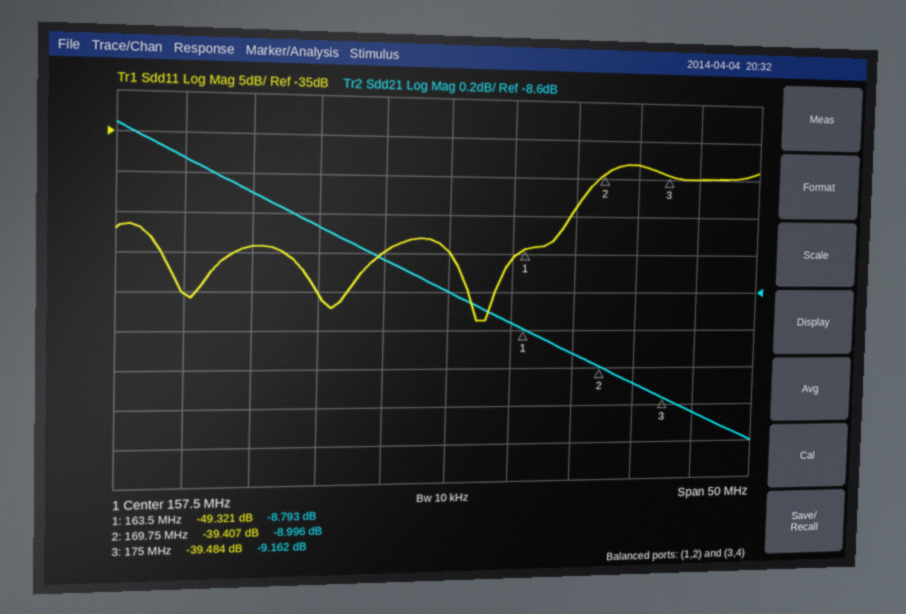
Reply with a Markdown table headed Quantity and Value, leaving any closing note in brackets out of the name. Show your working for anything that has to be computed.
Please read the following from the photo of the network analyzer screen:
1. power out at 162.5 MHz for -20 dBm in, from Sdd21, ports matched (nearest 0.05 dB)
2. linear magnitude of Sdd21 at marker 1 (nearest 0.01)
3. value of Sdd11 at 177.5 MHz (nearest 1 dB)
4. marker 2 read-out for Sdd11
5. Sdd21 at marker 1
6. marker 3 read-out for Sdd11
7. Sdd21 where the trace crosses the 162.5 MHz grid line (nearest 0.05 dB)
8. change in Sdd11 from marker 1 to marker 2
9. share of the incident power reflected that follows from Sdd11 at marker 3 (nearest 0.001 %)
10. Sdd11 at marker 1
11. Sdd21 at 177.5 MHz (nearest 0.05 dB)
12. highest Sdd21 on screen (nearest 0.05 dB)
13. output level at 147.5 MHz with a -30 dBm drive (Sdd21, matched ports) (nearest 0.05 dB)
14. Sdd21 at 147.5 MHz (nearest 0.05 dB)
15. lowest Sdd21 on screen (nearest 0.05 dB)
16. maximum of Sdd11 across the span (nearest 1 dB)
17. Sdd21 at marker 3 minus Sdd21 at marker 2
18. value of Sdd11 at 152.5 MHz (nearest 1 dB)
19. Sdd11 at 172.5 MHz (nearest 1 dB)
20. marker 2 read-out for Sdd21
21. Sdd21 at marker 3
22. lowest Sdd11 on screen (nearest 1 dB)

| Quantity | Value |
|---|---|
| power out at 162.5 MHz for -20 dBm in, from Sdd21, ports matched | -20 dBm + (-8.75 dB) = -28.75 dBm |
| linear magnitude of Sdd21 at marker 1 | 10^(-8.793/20) ≈ 0.36 |
| value of Sdd11 at 177.5 MHz | -40 dB |
| marker 2 read-out for Sdd11 | -39.407 dB |
| Sdd21 at marker 1 | -8.793 dB |
| marker 3 read-out for Sdd11 | -39.484 dB |
| Sdd21 where the trace crosses the 162.5 MHz grid line | -8.75 dB |
| change in Sdd11 from marker 1 to marker 2 | -39.407 − (-49.321) = 9.914 dB |
| share of the incident power reflected that follows from Sdd11 at marker 3 | 10^(-39.484/10) ≈ 0.011 % |
| Sdd11 at marker 1 | -49.321 dB |
| Sdd21 at 177.5 MHz | -9.25 dB |
| highest Sdd21 on screen | -7.75 dB |
| output level at 147.5 MHz with a -30 dBm drive (Sdd21, matched ports) | -30 dBm + (-8.25 dB) = -38.25 dBm |
| Sdd21 at 147.5 MHz | -8.25 dB |
| lowest Sdd21 on screen | -9.40 dB |
| maximum of Sdd11 across the span | -38 dB |
| Sdd21 at marker 3 minus Sdd21 at marker 2 | -9.162 − (-8.996) = -0.166 dB |
| value of Sdd11 at 152.5 MHz | -50 dB |
| Sdd11 at 172.5 MHz | -38 dB |
| marker 2 read-out for Sdd21 | -8.996 dB |
| Sdd21 at marker 3 | -9.162 dB |
| lowest Sdd11 on screen | -59 dB |
